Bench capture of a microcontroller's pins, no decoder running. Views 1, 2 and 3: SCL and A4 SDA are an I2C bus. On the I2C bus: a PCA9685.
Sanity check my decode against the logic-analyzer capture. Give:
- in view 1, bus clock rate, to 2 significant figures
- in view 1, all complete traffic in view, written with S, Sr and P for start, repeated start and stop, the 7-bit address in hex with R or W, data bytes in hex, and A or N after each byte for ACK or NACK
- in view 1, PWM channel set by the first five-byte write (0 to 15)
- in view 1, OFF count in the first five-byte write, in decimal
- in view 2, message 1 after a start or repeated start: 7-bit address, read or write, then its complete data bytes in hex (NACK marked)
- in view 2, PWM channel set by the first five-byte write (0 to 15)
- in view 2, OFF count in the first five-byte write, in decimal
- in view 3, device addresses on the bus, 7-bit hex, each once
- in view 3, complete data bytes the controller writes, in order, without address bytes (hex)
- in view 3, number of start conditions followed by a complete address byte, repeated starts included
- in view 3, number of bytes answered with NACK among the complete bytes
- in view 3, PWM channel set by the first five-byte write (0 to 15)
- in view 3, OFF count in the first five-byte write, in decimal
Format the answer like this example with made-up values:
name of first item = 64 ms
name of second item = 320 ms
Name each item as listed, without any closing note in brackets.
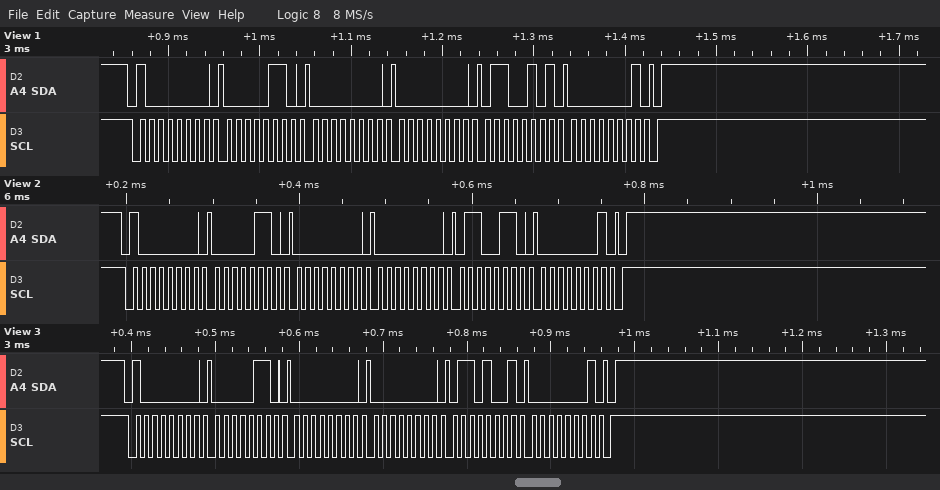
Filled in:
in view 1, bus clock rate, to 2 significant figures = 100 kHz
in view 1, all complete traffic in view, written with S, Sr and P for start, repeated start and stop, the 7-bit address in hex with R or W, data bytes in hex, and A or N after each byte for ACK or NACK = S 40W A 06 A 00 A 00 A 65 A 01 A P
in view 1, PWM channel set by the first five-byte write = 0
in view 1, OFF count in the first five-byte write, in decimal = 357
in view 2, message 1 after a start or repeated start: 7-bit address, read or write, then its complete data bytes in hex = 0x40 write: 06 00 00 66 01
in view 2, PWM channel set by the first five-byte write = 0
in view 2, OFF count in the first five-byte write, in decimal = 358
in view 3, device addresses on the bus, 7-bit hex, each once = 0x40
in view 3, complete data bytes the controller writes, in order, without address bytes = 06 00 00 69 01
in view 3, number of start conditions followed by a complete address byte, repeated starts included = 1
in view 3, number of bytes answered with NACK among the complete bytes = 0
in view 3, PWM channel set by the first five-byte write = 0
in view 3, OFF count in the first five-byte write, in decimal = 361
